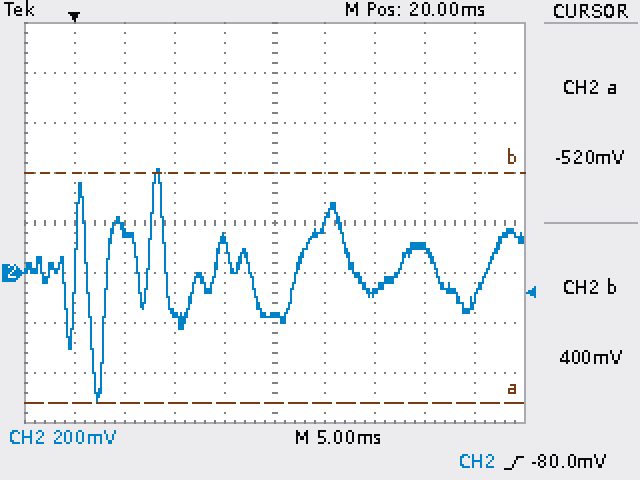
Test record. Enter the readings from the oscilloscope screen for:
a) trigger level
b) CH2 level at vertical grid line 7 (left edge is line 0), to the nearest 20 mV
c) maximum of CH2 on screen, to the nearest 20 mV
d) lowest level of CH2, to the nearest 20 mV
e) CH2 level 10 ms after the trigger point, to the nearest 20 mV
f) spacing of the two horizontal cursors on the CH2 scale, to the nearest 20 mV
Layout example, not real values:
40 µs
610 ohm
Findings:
-80.0 mV
-80 mV
420 mV
-520 mV
-160 mV
920 mV
